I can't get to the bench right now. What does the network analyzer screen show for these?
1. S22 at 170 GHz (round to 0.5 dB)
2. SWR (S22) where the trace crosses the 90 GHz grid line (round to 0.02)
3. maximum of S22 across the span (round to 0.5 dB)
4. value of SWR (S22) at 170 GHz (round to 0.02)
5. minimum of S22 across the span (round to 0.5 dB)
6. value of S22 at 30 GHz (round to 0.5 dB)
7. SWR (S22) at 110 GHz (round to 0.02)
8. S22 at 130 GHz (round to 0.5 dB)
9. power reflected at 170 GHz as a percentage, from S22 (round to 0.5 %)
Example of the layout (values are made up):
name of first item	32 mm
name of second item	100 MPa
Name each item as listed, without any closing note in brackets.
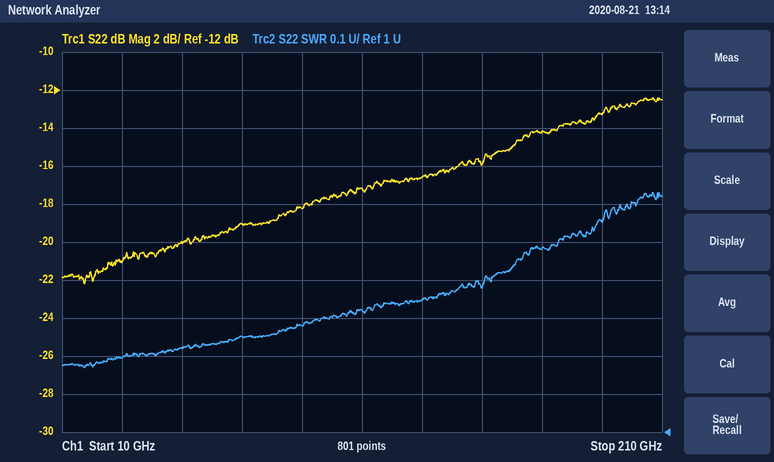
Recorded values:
S22 at 170 GHz	-14.0 dB
SWR (S22) where the trace crosses the 90 GHz grid line	1.28
maximum of S22 across the span	-12.5 dB
value of SWR (S22) at 170 GHz	1.48
minimum of S22 across the span	-22.0 dB
value of S22 at 30 GHz	-21.0 dB
SWR (S22) at 110 GHz	1.32
S22 at 130 GHz	-16.5 dB
power reflected at 170 GHz as a percentage, from S22	4.0 %
